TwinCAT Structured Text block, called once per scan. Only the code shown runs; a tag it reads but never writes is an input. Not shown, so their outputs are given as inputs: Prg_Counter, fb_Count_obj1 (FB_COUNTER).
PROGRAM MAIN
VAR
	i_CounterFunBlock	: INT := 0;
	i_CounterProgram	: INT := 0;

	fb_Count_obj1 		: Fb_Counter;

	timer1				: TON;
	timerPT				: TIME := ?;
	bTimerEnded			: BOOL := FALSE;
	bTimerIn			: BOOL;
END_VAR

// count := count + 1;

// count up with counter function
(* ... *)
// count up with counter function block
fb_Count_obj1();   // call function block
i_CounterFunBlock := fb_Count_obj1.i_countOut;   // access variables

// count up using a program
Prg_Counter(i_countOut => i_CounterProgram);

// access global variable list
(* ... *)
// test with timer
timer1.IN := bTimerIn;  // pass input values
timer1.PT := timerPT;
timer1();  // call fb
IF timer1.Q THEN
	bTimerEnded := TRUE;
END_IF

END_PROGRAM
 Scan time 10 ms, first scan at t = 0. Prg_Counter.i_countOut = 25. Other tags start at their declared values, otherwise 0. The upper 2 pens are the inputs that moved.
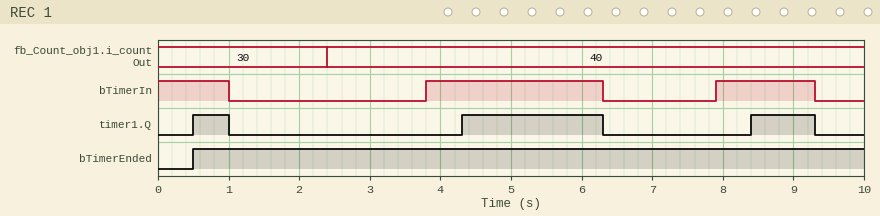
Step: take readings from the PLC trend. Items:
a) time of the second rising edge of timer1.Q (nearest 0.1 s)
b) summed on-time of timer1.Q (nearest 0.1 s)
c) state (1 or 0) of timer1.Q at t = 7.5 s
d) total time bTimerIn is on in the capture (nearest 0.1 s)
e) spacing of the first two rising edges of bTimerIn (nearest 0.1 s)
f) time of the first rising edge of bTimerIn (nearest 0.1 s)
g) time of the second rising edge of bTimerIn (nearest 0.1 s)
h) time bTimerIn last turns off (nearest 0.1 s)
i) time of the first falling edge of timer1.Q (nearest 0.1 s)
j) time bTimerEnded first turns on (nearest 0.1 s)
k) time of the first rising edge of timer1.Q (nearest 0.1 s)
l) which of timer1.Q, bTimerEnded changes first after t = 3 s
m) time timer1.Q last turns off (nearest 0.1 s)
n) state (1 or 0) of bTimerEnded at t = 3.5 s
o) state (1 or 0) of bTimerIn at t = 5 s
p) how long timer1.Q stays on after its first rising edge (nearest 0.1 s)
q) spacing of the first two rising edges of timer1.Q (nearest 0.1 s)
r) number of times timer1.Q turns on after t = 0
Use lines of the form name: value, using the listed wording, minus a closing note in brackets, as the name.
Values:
time of the second rising edge of timer1.Q: 4.3 s
summed on-time of timer1.Q: 3.4 s
state (1 or 0) of timer1.Q at t = 7.5 s: 0
total time bTimerIn is on in the capture: 4.9 s
spacing of the first two rising edges of bTimerIn: 4.1 s
time of the first rising edge of bTimerIn: 3.8 s
time of the second rising edge of bTimerIn: 7.9 s
time bTimerIn last turns off: 9.3 s
time of the first falling edge of timer1.Q: 1.0 s
time bTimerEnded first turns on: 0.5 s
time of the first rising edge of timer1.Q: 0.5 s
which of timer1.Q, bTimerEnded changes first after t = 3 s: timer1.Q
time timer1.Q last turns off: 9.3 s
state (1 or 0) of bTimerEnded at t = 3.5 s: 1
state (1 or 0) of bTimerIn at t = 5 s: 1
how long timer1.Q stays on after its first rising edge: 0.5 s
spacing of the first two rising edges of timer1.Q: 3.8 s
number of times timer1.Q turns on after t = 0: 3
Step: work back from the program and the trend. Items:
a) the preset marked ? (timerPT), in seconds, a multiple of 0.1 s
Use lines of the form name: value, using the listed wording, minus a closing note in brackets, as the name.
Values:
the preset marked ? (timerPT), in seconds, a multiple of 0.1 s: 0.5 s
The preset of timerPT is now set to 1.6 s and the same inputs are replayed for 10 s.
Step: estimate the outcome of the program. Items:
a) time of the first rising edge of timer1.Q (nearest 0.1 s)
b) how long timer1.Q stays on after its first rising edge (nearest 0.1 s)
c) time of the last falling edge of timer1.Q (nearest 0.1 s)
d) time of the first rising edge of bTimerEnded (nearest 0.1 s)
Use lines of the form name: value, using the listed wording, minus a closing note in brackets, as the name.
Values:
time of the first rising edge of timer1.Q: 5.4 s
how long timer1.Q stays on after its first rising edge: 0.9 s
time of the last falling edge of timer1.Q: 6.3 s
time of the first rising edge of bTimerEnded: 5.4 s
